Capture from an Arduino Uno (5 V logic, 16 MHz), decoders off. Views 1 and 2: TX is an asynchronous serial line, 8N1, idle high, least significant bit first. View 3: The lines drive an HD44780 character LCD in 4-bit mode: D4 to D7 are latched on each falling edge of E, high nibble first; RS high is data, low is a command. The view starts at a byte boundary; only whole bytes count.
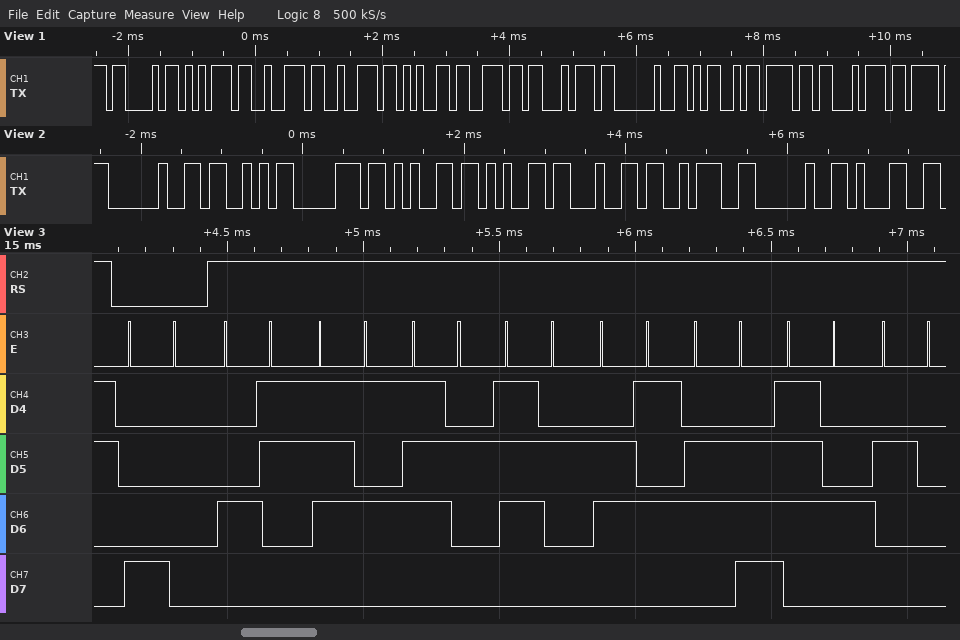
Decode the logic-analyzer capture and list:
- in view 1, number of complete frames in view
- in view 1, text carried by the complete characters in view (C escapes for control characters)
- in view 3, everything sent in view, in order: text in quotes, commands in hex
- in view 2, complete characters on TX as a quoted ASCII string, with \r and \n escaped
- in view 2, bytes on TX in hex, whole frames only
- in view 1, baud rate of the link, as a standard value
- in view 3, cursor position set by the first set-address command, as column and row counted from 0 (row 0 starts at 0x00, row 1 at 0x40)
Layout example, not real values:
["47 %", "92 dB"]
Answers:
["11", "\"Current Mot\"", "0x80 \"Current \"", "\" Speed: 1\"", "20 53 70 65 65 64 3A 20 31", "9600 baud", "column 0, row 0"]
